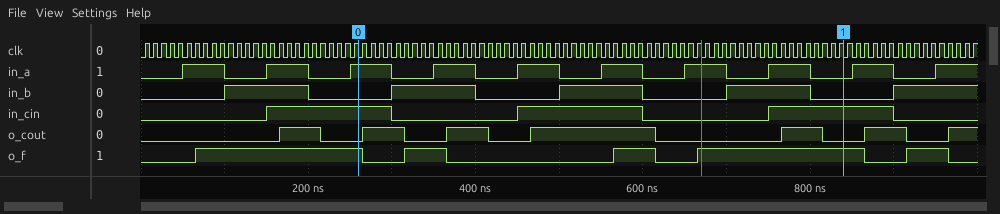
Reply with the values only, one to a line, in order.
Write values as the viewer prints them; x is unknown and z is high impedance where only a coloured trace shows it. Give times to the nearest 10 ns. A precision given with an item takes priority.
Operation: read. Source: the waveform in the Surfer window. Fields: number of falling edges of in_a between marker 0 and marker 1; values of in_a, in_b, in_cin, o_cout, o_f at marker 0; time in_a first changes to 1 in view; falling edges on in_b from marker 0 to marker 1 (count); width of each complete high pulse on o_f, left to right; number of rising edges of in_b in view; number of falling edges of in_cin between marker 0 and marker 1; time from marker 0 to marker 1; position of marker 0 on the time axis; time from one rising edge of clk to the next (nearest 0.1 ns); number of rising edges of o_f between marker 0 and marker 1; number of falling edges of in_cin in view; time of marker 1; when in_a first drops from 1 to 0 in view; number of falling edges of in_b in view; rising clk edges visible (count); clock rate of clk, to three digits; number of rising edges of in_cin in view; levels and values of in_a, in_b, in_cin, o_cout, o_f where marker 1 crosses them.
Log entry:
6
in_a=1, in_b=0, in_cin=1, o_cout=0, o_f=1
50 ns
3
200 ns, 50 ns, 50 ns, 200 ns, 50 ns
5
2
580 ns
260 ns
10 ns
3
3
840 ns
100 ns
4
100
100 MHz
3
in_a=0, in_b=0, in_cin=1, o_cout=0, o_f=1
